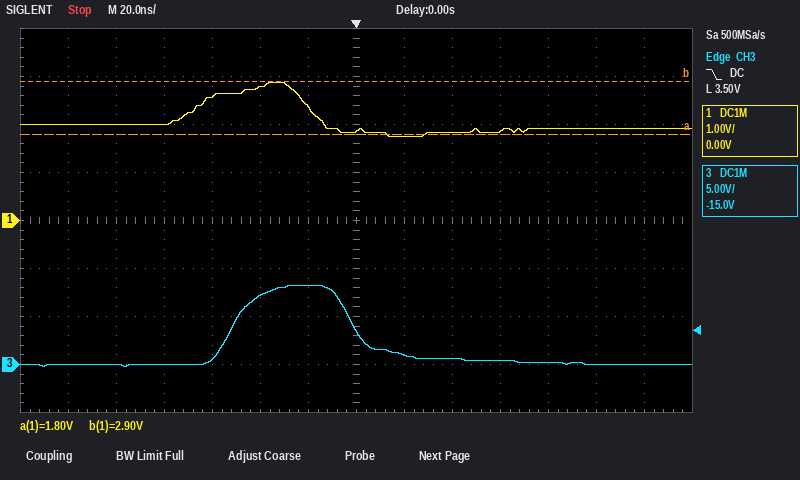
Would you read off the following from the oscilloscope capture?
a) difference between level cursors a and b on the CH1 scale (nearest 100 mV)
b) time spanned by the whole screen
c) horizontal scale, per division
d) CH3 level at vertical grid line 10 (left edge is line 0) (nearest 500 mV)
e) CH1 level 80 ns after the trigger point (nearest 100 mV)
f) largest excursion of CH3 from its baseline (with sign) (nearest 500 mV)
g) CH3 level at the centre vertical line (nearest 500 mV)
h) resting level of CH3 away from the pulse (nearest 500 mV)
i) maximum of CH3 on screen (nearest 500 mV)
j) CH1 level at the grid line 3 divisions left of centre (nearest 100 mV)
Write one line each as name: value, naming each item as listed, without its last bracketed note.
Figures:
difference between level cursors a and b on the CH1 scale: 1.1 V
time spanned by the whole screen: 280 ns
horizontal scale, per division: 20 ns
CH3 level at vertical grid line 10 (left edge is line 0): 500 mV
CH1 level 80 ns after the trigger point: 1.9 V
largest excursion of CH3 from its baseline (with sign): +8.0 V
CH3 level at the centre vertical line: 3.5 V
resting level of CH3 away from the pulse: 0.0 V
maximum of CH3 on screen: 8.0 V
CH1 level at the grid line 3 divisions left of centre: 2.6 V
